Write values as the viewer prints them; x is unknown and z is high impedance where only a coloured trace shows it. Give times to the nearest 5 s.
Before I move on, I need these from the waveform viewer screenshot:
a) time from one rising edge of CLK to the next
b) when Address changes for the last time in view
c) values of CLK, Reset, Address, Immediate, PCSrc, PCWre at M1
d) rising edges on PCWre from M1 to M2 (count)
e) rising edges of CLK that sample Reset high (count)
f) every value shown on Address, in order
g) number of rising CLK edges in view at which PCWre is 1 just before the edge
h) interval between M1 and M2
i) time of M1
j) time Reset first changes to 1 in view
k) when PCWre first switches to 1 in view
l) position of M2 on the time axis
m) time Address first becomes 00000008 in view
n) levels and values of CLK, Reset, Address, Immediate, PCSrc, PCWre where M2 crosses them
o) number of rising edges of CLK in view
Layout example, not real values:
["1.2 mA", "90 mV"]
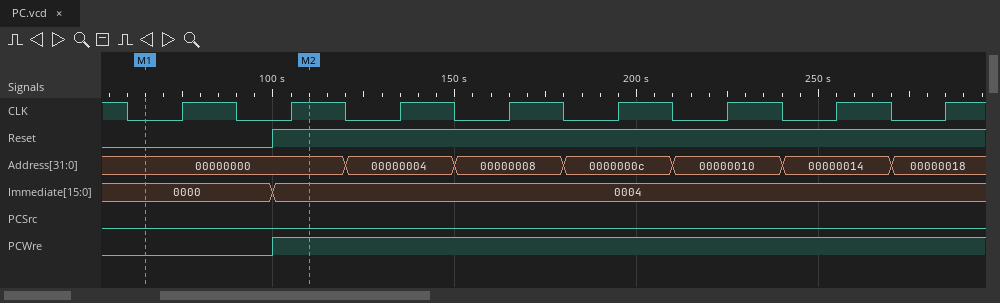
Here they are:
["30 s", "270 s", "CLK=0, Reset=0, Address=00000000, Immediate=0000, PCSrc=0, PCWre=0", "1", "7", "00000000, 00000004, 00000008, 0000000c, 00000010, 00000014, 00000018", "7", "45 s", "65 s", "100 s", "100 s", "110 s", "150 s", "CLK=1, Reset=1, Address=00000000, Immediate=0004, PCSrc=0, PCWre=1", "8"]
